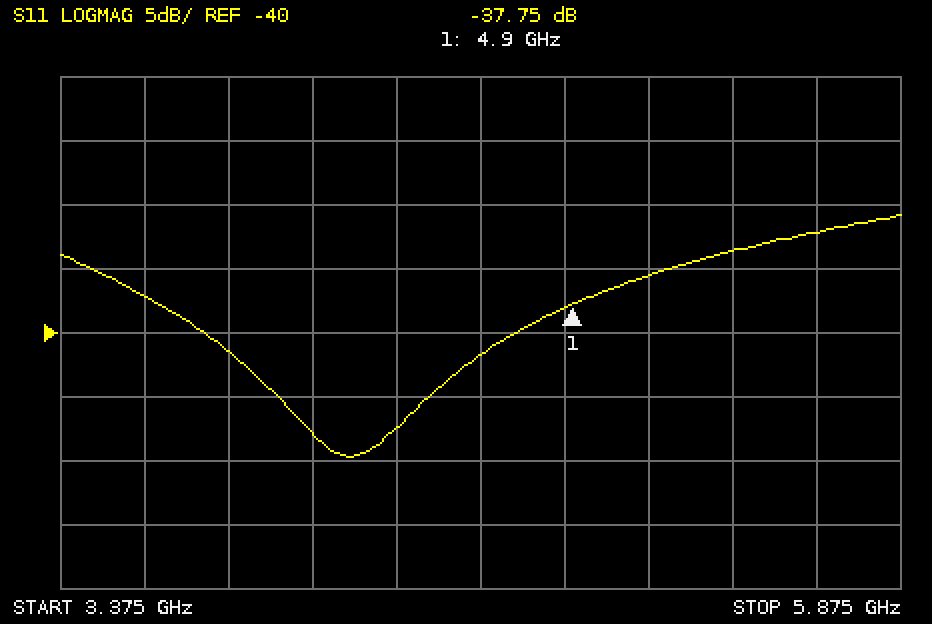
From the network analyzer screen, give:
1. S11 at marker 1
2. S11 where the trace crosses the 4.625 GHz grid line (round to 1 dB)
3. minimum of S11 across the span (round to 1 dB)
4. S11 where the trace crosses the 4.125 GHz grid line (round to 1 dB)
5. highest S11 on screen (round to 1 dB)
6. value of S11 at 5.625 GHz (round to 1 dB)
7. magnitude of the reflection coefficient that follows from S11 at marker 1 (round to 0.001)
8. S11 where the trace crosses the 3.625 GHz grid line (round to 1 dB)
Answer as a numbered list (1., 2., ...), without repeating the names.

1. -37.75 dB
2. -42 dB
3. -50 dB
4. -48 dB
5. -31 dB
6. -32 dB
7. 0.013
8. -37 dB
